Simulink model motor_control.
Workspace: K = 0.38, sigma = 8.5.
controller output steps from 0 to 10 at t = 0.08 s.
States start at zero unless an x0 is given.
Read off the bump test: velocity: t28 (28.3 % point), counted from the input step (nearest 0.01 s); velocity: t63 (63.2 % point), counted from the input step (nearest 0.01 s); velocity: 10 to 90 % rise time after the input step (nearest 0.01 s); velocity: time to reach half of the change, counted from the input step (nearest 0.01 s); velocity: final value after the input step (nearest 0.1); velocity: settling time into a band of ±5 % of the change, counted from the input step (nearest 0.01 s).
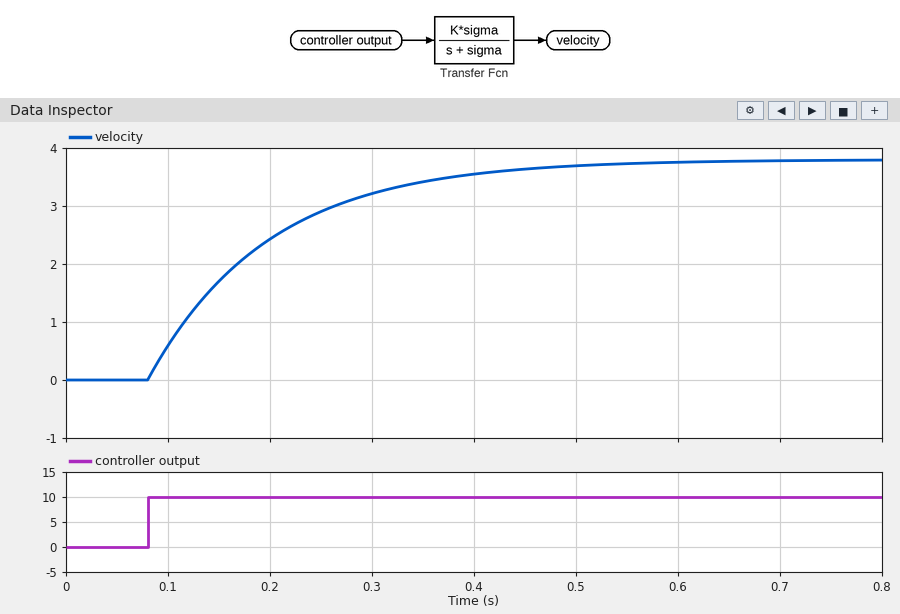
0.04 s
0.12 s
0.26 s
0.08 s
3.8
0.35 s
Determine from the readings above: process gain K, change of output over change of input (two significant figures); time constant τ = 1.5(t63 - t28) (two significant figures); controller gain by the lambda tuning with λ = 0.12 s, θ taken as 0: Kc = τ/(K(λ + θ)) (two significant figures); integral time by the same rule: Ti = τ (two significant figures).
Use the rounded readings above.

0.38
0.12 s
2.6
0.12 s
